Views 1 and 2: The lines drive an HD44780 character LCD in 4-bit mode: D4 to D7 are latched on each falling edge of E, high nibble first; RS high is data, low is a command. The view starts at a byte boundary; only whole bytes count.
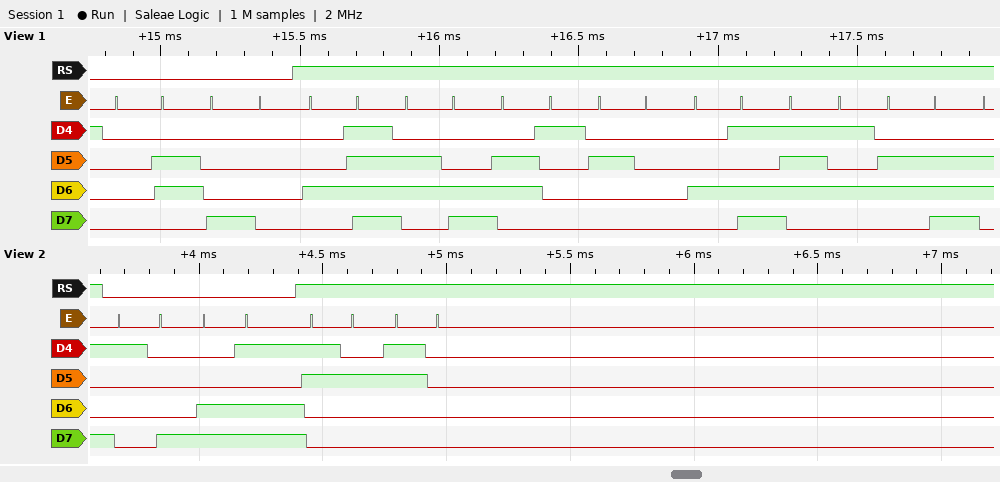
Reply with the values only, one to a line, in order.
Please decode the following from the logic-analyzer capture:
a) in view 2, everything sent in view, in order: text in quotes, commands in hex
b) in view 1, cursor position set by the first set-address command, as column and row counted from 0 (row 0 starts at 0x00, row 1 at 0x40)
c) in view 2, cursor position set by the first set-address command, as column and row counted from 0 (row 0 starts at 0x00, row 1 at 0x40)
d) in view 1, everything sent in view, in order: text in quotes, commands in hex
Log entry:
0x18 0xCD "20"
column 0, row 0
column 13, row 1
0x06 0x80 "Ola Mun"
